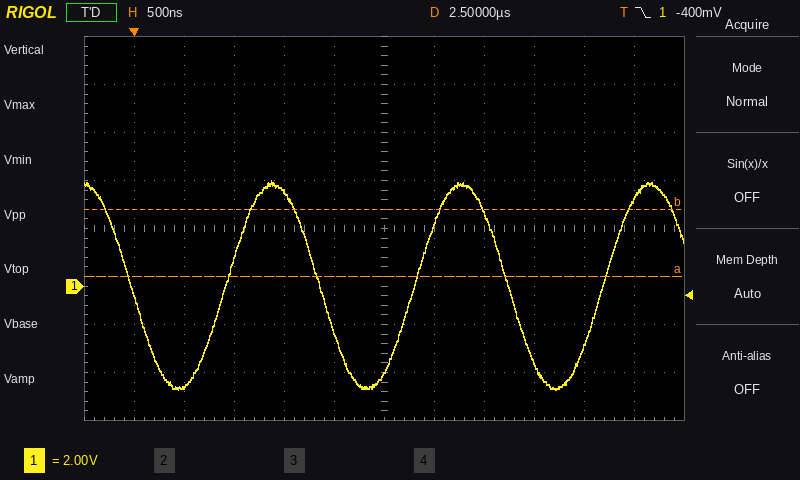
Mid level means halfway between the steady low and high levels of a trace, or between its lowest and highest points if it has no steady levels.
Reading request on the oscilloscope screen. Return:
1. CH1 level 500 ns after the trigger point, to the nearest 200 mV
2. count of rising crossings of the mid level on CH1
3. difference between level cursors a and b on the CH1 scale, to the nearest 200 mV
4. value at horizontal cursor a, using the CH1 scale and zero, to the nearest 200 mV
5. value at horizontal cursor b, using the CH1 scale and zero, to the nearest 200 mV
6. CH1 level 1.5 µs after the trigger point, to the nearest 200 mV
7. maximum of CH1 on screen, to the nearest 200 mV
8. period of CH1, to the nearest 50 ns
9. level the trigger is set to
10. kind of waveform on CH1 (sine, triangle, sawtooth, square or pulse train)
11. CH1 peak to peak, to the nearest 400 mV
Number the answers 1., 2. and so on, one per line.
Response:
1. -4.2 V
2. 3
3. 2.8 V
4. 400 mV
5. 3.2 V
6. 4.0 V
7. 4.4 V
8. 1.90 µs
9. -400 mV
10. sine
11. 8.8 V
